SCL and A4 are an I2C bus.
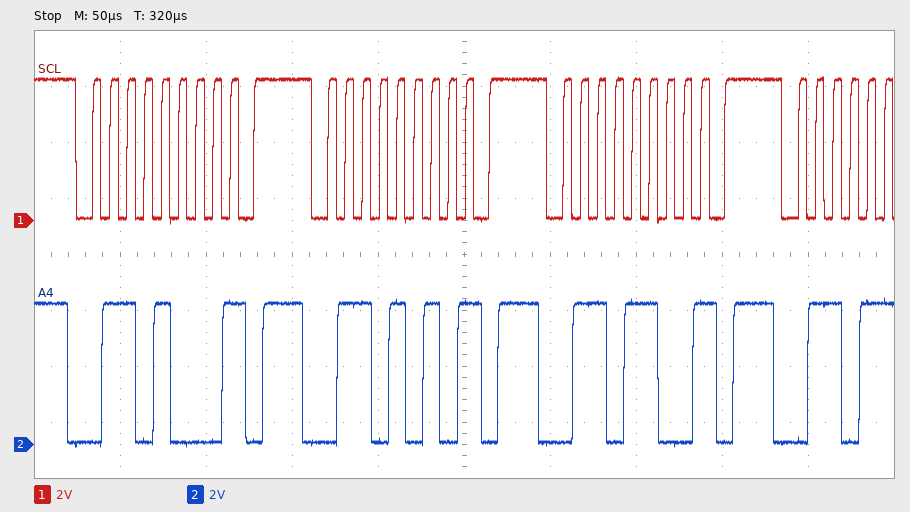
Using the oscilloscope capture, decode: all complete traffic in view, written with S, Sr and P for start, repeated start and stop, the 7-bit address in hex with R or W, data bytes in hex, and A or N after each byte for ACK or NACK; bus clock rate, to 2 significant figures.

S 34W N P S 35W N P S 36W N P
100 kHz
